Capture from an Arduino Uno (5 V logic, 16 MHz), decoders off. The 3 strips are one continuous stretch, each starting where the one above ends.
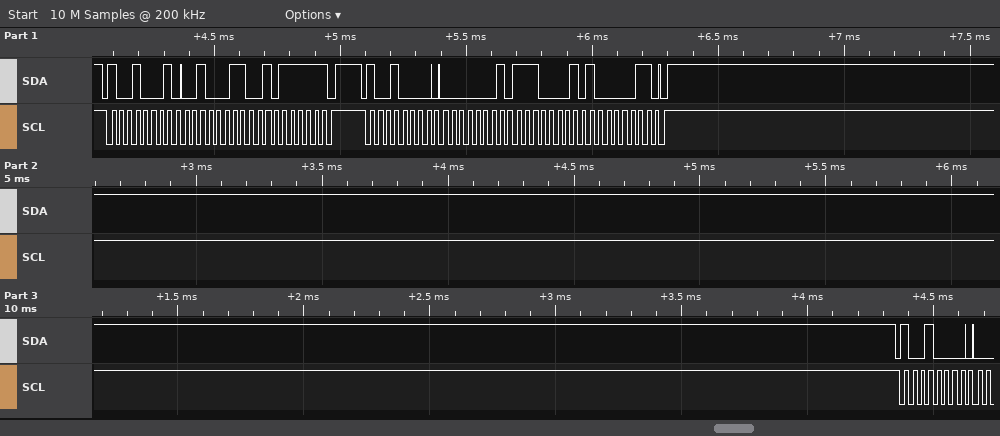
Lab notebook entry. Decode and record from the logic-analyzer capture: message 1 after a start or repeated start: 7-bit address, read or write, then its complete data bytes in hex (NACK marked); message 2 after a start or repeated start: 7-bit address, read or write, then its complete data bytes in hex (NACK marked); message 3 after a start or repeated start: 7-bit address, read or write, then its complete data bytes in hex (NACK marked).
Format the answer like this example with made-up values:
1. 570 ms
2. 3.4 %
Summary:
1. 0x48 read: 23 5F NACK
2. 0x48 write: 01 E1 83
3. 0x48 write
